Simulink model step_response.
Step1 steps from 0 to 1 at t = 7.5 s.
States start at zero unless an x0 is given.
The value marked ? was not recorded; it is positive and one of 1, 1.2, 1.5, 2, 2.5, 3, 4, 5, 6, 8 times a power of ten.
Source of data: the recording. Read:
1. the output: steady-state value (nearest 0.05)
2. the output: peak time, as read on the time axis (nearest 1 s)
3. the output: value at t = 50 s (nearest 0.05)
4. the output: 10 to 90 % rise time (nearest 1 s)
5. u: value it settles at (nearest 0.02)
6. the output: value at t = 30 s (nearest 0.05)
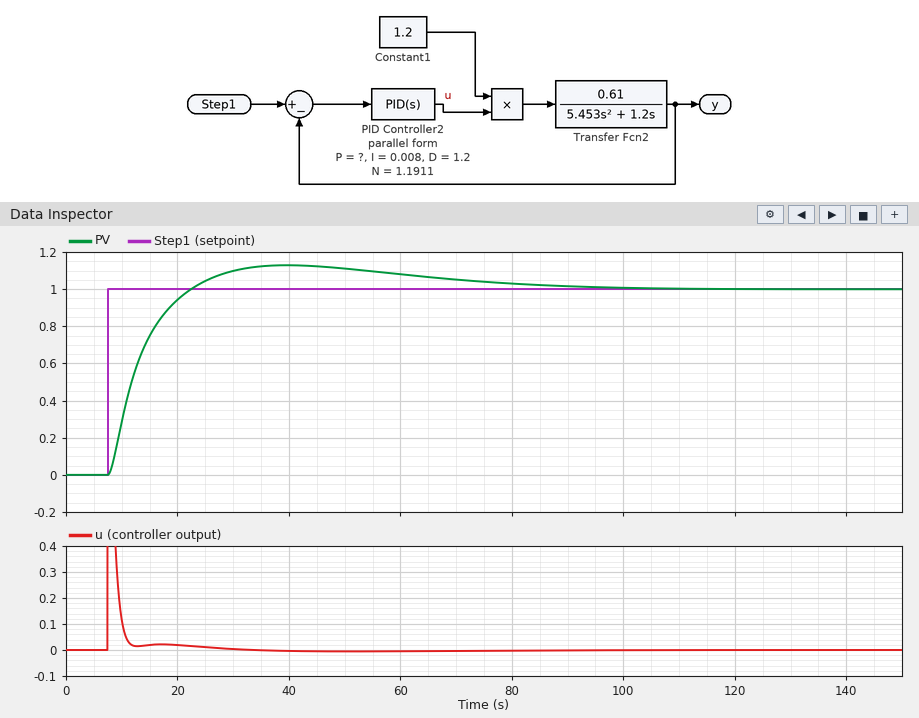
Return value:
1.00
40 s
1.10
10 s
0.00
1.10
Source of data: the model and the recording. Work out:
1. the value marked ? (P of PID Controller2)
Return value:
0.25
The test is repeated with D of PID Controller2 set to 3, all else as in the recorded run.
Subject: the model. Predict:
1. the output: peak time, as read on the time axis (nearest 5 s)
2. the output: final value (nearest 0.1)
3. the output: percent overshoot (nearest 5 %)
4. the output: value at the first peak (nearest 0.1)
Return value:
55 s
1.0
10 %
1.1
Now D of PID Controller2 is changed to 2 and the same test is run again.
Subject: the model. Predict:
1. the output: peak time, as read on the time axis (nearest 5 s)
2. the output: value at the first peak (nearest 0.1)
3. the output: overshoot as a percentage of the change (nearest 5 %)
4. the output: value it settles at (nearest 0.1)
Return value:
50 s
1.1
10 %
1.0
